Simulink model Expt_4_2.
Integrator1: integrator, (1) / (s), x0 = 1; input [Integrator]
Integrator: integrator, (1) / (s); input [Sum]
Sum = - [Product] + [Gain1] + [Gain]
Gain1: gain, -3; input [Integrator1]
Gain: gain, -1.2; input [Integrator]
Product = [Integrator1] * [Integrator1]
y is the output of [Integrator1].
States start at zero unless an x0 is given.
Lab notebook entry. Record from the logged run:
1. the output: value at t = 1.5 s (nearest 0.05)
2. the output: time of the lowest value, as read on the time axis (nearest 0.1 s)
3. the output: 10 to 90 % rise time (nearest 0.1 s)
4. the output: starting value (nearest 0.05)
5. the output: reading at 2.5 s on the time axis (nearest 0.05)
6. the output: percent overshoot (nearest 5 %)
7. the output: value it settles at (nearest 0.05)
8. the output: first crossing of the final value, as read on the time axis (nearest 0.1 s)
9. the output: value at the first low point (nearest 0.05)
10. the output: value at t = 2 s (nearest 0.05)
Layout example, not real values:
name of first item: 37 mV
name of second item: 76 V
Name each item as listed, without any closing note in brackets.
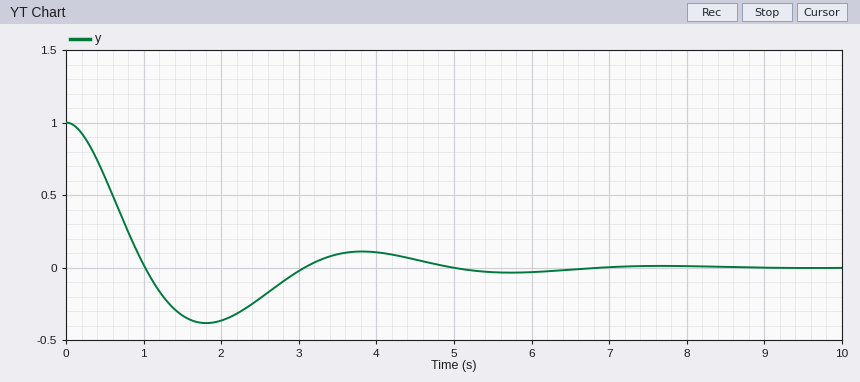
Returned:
the output: value at t = 1.5 s: -0.35
the output: time of the lowest value, as read on the time axis: 1.8 s
the output: 10 to 90 % rise time: 0.7 s
the output: starting value: 1.00
the output: reading at 2.5 s on the time axis: -0.20
the output: percent overshoot: 40 %
the output: value it settles at: 0.00
the output: first crossing of the final value, as read on the time axis: 1.0 s
the output: value at the first low point: -0.40
the output: value at t = 2 s: -0.35
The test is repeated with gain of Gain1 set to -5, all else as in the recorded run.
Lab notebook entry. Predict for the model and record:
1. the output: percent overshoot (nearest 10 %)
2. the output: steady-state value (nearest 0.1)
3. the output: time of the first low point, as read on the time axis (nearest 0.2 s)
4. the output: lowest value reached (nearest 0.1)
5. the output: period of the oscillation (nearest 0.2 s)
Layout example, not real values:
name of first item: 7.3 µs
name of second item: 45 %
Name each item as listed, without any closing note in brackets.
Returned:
the output: percent overshoot: 50 %
the output: steady-state value: 0.0
the output: time of the first low point, as read on the time axis: 1.4 s
the output: lowest value reached: -0.5
the output: period of the oscillation: 3.0 s
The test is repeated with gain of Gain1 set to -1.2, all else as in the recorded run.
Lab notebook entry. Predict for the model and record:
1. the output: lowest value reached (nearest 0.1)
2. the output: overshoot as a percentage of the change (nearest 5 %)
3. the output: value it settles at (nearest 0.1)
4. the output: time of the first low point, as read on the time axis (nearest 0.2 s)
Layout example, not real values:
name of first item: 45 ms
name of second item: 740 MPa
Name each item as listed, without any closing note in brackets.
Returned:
the output: lowest value reached: -0.2
the output: overshoot as a percentage of the change: 25 %
the output: value it settles at: 0.0
the output: time of the first low point, as read on the time axis: 2.8 s
